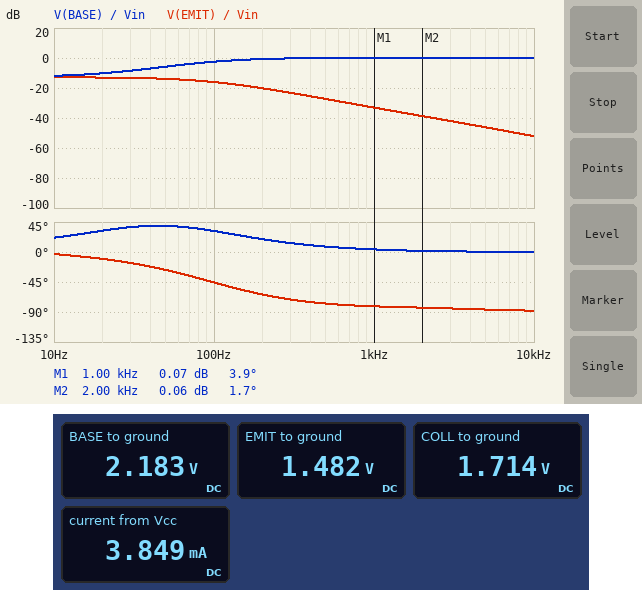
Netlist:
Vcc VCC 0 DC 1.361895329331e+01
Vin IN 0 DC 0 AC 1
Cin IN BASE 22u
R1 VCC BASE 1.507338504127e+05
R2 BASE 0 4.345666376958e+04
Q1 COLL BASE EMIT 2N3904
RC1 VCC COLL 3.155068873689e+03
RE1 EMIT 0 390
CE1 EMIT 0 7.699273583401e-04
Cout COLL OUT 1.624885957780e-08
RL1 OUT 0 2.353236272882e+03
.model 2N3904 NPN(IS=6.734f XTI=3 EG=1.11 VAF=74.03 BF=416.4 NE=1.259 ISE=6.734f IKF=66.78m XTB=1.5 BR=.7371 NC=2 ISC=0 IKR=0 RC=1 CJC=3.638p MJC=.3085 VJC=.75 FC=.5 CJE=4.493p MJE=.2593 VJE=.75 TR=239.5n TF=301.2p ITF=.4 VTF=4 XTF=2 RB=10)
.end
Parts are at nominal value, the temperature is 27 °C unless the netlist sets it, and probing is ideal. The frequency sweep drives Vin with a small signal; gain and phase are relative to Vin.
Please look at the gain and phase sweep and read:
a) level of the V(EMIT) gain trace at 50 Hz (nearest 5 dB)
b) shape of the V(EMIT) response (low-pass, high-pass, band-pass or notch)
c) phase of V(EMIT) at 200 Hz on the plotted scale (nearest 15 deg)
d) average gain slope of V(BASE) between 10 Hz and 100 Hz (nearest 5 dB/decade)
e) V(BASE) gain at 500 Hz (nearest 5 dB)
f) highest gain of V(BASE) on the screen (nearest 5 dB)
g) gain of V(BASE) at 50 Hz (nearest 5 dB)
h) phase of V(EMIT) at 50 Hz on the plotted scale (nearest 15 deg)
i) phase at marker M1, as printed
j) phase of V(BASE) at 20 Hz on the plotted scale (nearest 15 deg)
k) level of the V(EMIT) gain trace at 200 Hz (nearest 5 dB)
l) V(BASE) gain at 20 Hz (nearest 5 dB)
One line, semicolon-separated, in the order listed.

-15 dB; low-pass; -60 deg; 10 dB/decade; 0 dB; 0 dB; -5 dB; -30 deg; 3.9 deg; 30 deg; -20 dB; -10 dB
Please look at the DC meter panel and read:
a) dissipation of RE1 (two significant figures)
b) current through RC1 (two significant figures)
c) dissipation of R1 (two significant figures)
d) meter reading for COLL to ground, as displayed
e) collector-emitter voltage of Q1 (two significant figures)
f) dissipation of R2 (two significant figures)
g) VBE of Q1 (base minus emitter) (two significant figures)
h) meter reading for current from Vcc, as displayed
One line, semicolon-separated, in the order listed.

5.6 mW; 3.8 mA; 870 µW; 1.714 V; 230 mV; 110 µW; 700 mV; 3.849 mA
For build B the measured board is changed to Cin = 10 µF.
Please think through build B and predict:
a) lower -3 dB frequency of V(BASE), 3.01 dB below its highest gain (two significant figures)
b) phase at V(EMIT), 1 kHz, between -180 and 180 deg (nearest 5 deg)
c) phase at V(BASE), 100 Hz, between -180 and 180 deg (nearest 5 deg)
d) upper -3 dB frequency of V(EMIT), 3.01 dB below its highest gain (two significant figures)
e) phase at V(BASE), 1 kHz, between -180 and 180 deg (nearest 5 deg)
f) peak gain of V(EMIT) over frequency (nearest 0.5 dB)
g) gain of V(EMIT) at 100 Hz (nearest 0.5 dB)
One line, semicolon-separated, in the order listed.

180 Hz; -75 deg; 50 deg; 190 Hz; 10 deg; -18.5 dB; -19.5 dB
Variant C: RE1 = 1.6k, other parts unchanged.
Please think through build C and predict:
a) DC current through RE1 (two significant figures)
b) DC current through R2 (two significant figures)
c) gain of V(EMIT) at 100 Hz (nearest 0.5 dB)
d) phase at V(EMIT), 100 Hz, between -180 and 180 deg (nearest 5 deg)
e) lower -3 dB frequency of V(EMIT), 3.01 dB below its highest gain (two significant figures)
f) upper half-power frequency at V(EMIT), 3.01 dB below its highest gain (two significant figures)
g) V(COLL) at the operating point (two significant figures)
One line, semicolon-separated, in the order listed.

1.3 mA; 63 µA; -20.5 dB; -85 deg; 190 mHz; 12 Hz; 9.5 V
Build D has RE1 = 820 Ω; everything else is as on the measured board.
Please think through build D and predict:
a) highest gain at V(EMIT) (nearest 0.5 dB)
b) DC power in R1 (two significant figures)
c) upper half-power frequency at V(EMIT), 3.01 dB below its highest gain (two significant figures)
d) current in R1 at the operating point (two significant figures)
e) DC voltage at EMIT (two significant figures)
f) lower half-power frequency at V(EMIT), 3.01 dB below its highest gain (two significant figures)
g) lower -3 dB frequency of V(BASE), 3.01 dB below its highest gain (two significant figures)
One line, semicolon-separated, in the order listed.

-2.0 dB; 810 µW; 20 Hz; 73 µA; 1.9 V; 220 mHz; 380 mHz
